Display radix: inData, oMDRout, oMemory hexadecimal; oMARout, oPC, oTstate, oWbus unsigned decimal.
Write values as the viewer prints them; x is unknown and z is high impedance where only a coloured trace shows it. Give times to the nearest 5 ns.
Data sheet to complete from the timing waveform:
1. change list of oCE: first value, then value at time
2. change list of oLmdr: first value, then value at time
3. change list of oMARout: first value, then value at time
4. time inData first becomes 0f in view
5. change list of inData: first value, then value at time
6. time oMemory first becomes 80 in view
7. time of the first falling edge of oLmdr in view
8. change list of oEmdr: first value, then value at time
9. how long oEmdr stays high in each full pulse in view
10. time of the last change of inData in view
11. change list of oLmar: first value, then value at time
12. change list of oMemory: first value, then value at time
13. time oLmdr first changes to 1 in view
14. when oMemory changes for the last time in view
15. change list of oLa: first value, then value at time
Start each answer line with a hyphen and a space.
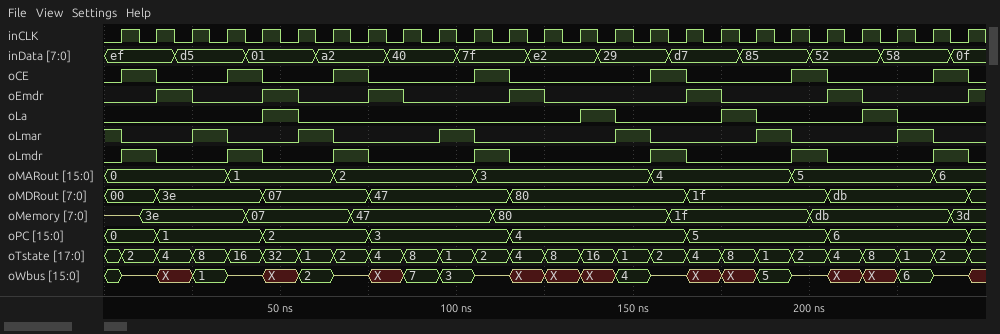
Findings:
- 0, 1 at 5 ns, 0 at 15 ns, 1 at 35 ns, 0 at 45 ns, 1 at 65 ns, 0 at 75 ns, 1 at 105 ns, 0 at 115 ns, 1 at 155 ns, 0 at 165 ns, 1 at 195 ns, 0 at 205 ns, 1 at 235 ns, 0 at 245 ns
- 0, 1 at 5 ns, 0 at 15 ns, 1 at 35 ns, 0 at 45 ns, 1 at 65 ns, 0 at 75 ns, 1 at 105 ns, 0 at 115 ns, 1 at 155 ns, 0 at 165 ns, 1 at 195 ns, 0 at 205 ns, 1 at 235 ns, 0 at 245 ns
- 0, 1 at 35 ns, 2 at 65 ns, 3 at 105 ns, 4 at 155 ns, 5 at 195 ns, 6 at 235 ns
- 240 ns
- ef, d5 at 20 ns, 01 at 40 ns, a2 at 60 ns, 40 at 80 ns, 7f at 100 ns, e2 at 120 ns, 29 at 140 ns, d7 at 160 ns, 85 at 180 ns, 52 at 200 ns, 58 at 220 ns, 0f at 240 ns
- 110 ns
- 15 ns
- 0, 1 at 15 ns, 0 at 25 ns, 1 at 45 ns, 0 at 55 ns, 1 at 75 ns, 0 at 85 ns, 1 at 115 ns, 0 at 125 ns, 1 at 165 ns, 0 at 175 ns, 1 at 205 ns, 0 at 215 ns, 1 at 245 ns
- 10 ns, 10 ns, 10 ns, 10 ns, 10 ns, 10 ns
- 240 ns
- 1, 0 at 5 ns, 1 at 25 ns, 0 at 35 ns, 1 at 55 ns, 0 at 65 ns, 1 at 95 ns, 0 at 105 ns, 1 at 145 ns, 0 at 155 ns, 1 at 185 ns, 0 at 195 ns, 1 at 225 ns, 0 at 235 ns
- z, 3e at 10 ns, 07 at 40 ns, 47 at 70 ns, 80 at 110 ns, 1f at 160 ns, db at 200 ns, 3d at 240 ns
- 5 ns
- 240 ns
- 0, 1 at 45 ns, 0 at 55 ns, 1 at 135 ns, 0 at 145 ns, 1 at 175 ns, 0 at 185 ns, 1 at 215 ns, 0 at 225 ns
